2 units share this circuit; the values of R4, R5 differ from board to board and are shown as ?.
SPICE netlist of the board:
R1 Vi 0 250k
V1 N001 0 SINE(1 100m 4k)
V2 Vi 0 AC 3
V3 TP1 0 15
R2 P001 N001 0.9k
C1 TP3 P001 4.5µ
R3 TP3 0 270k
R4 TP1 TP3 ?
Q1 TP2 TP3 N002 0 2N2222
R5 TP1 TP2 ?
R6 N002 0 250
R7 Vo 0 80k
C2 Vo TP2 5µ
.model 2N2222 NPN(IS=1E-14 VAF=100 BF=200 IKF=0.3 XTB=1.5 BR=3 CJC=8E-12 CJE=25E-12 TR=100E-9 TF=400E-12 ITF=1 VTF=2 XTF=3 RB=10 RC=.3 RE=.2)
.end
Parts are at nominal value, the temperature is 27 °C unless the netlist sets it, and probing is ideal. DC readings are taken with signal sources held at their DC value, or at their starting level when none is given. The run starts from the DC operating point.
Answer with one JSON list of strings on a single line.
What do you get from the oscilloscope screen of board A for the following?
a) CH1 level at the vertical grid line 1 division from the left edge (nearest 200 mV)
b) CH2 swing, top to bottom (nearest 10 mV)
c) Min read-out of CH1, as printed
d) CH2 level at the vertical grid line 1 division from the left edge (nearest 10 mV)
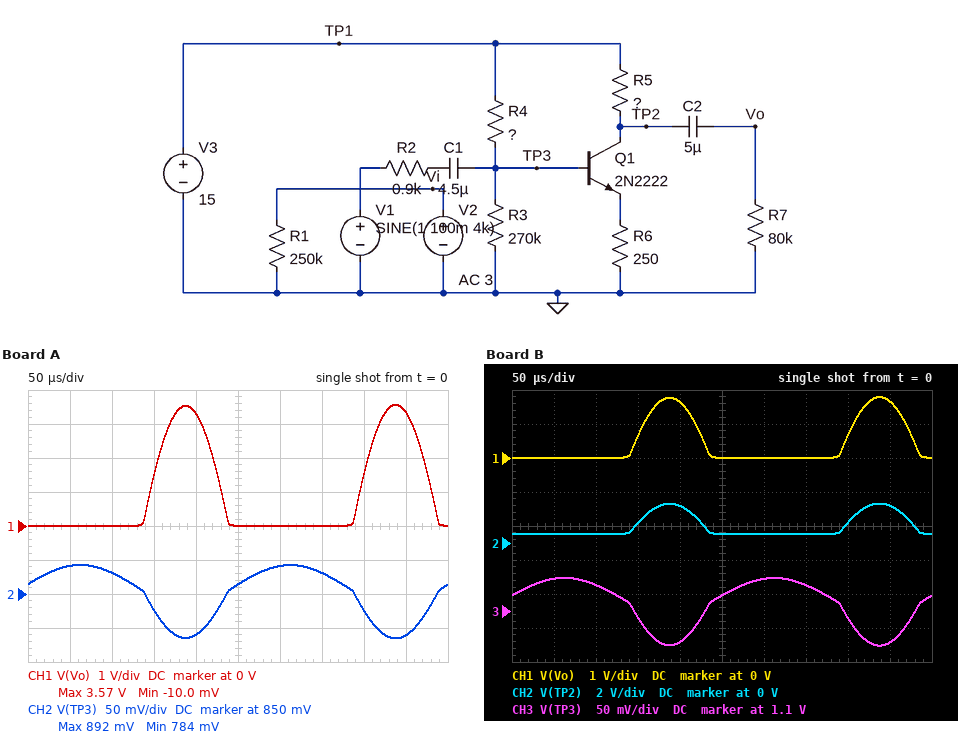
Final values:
["0 V", "110 mV", "-10.0 mV", "890 mV"]
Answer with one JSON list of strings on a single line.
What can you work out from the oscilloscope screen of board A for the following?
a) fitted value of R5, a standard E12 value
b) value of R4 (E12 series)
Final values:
["18 kΩ", "470 kΩ"]
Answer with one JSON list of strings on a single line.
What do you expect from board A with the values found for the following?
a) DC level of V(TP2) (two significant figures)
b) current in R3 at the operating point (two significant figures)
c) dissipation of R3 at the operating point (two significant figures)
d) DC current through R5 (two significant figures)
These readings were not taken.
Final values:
["280 mV", "3.2 µA", "2.8 µW", "820 µA"]
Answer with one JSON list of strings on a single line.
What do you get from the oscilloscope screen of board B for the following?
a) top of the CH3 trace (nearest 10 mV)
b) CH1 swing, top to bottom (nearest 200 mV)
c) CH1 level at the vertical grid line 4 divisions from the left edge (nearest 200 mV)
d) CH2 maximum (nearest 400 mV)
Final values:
["1.15 V", "1.8 V", "1.6 V", "2.4 V"]
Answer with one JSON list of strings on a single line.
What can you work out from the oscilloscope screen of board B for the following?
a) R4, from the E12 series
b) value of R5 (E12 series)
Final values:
["330 kΩ", "8.2 kΩ"]
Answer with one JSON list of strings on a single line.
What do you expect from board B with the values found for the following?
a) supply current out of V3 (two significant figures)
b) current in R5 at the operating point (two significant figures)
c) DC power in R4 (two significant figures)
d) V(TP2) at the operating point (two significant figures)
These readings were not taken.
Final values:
["1.8 mA", "1.8 mA", "580 µW", "530 mV"]
